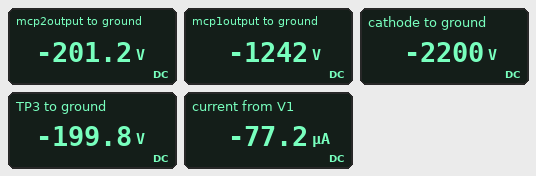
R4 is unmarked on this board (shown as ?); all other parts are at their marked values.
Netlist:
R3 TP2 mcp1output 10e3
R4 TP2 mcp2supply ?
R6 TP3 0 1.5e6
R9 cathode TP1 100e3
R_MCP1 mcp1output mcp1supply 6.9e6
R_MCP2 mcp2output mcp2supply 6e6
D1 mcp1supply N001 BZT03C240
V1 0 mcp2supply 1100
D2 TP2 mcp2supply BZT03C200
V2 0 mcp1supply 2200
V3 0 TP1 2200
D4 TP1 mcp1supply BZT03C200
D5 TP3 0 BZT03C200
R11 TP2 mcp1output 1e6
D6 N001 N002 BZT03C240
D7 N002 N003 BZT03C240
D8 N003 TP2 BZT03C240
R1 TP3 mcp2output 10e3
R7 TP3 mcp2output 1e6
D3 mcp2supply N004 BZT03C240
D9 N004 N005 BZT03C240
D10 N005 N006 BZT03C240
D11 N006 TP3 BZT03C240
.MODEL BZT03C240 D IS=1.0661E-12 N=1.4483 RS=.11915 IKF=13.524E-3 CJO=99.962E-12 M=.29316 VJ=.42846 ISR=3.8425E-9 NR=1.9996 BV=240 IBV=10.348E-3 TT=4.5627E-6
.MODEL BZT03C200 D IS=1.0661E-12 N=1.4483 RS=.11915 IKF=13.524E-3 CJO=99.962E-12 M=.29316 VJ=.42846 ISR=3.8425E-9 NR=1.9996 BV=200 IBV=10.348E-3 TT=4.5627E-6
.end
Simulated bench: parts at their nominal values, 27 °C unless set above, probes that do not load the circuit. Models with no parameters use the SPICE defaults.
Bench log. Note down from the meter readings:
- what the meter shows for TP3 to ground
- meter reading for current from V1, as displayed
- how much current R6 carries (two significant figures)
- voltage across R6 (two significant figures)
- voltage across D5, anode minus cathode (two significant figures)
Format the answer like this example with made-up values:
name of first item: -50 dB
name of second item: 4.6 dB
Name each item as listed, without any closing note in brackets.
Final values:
what the meter shows for TP3 to ground: -199.8 V
meter reading for current from V1, as displayed: -77.2 µA
how much current R6 carries: 130 µA
voltage across R6: 200 V
voltage across D5, anode minus cathode: -200 V
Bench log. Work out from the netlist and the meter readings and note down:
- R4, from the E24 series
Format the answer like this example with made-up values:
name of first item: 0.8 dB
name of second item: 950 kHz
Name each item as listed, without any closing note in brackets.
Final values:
R4, from the E24 series: 620 kΩ
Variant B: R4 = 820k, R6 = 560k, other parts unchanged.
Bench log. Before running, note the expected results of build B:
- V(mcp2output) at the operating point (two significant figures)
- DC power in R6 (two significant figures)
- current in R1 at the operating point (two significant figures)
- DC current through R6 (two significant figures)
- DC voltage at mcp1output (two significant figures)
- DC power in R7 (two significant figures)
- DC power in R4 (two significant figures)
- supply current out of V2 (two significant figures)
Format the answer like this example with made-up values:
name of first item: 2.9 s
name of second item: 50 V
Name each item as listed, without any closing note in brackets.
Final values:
V(mcp2output) at the operating point: -140 V
DC power in R6: 35 mW
current in R1 at the operating point: 160 µA
DC current through R6: 250 µA
DC voltage at mcp1output: -1.2 kV
DC power in R7: 2.5 µW
DC power in R4: 24 mW
supply current out of V2: 170 µA
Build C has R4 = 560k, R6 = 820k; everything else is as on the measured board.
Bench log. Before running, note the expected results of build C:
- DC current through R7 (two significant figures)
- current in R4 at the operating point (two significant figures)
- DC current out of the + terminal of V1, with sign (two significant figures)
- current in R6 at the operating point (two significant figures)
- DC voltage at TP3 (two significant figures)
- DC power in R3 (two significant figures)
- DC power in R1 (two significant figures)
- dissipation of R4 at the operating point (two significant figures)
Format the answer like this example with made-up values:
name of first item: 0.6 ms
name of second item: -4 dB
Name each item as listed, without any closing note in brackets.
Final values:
DC current through R7: 1.6 µA
current in R4 at the operating point: 250 µA
DC current out of the + terminal of V1, with sign: -79 µA
current in R6 at the operating point: 170 µA
DC voltage at TP3: -140 V
DC power in R3: 190 µW
DC power in R1: 250 µW
dissipation of R4 at the operating point: 35 mW
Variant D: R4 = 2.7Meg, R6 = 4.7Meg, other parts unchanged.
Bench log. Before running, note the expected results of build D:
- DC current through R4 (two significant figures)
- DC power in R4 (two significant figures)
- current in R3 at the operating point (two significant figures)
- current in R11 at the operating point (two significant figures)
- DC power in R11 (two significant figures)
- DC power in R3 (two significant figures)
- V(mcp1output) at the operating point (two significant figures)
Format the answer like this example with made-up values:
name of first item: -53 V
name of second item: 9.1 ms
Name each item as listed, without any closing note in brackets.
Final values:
DC current through R4: 74 µA
DC power in R4: 15 mW
current in R3 at the operating point: 130 µA
current in R11 at the operating point: 1.3 µA
DC power in R11: 1.7 µW
DC power in R3: 170 µW
V(mcp1output) at the operating point: -1.3 kV
